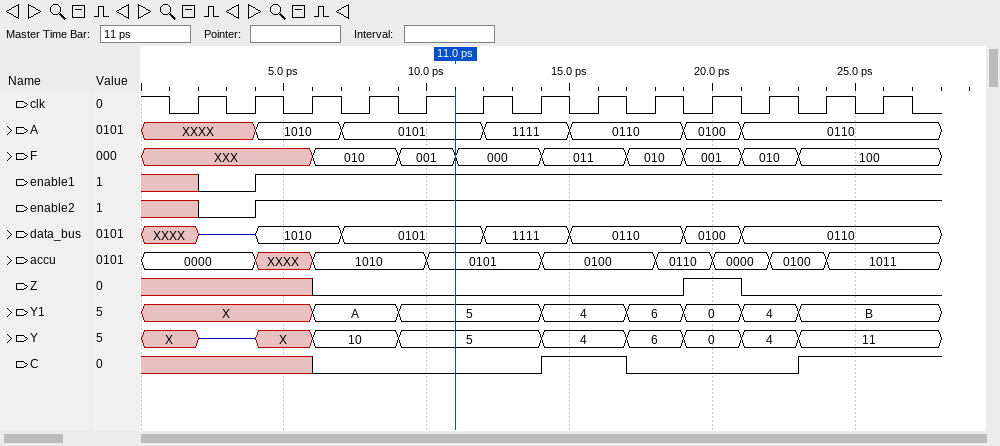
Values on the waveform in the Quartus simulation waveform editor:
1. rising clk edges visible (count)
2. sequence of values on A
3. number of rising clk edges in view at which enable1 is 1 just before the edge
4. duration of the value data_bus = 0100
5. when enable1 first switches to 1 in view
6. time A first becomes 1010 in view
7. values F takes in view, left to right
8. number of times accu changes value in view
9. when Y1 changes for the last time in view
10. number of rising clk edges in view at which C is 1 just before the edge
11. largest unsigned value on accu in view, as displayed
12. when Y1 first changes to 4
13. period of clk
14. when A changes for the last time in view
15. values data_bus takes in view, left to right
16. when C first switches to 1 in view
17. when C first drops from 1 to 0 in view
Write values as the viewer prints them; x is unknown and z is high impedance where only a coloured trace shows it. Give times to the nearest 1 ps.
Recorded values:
13
XXXX, 1010, 0101, 1111, 0110, 0100, 0110
11
2 ps
4 ps
4 ps
XXX, 010, 001, 000, 011, 010, 001, 010, 100
8
23 ps
3
1011
14 ps
2 ps
21 ps
XXXX, z, 1010, 0101, 1111, 0110, 0100, 0110
14 ps
17 ps
